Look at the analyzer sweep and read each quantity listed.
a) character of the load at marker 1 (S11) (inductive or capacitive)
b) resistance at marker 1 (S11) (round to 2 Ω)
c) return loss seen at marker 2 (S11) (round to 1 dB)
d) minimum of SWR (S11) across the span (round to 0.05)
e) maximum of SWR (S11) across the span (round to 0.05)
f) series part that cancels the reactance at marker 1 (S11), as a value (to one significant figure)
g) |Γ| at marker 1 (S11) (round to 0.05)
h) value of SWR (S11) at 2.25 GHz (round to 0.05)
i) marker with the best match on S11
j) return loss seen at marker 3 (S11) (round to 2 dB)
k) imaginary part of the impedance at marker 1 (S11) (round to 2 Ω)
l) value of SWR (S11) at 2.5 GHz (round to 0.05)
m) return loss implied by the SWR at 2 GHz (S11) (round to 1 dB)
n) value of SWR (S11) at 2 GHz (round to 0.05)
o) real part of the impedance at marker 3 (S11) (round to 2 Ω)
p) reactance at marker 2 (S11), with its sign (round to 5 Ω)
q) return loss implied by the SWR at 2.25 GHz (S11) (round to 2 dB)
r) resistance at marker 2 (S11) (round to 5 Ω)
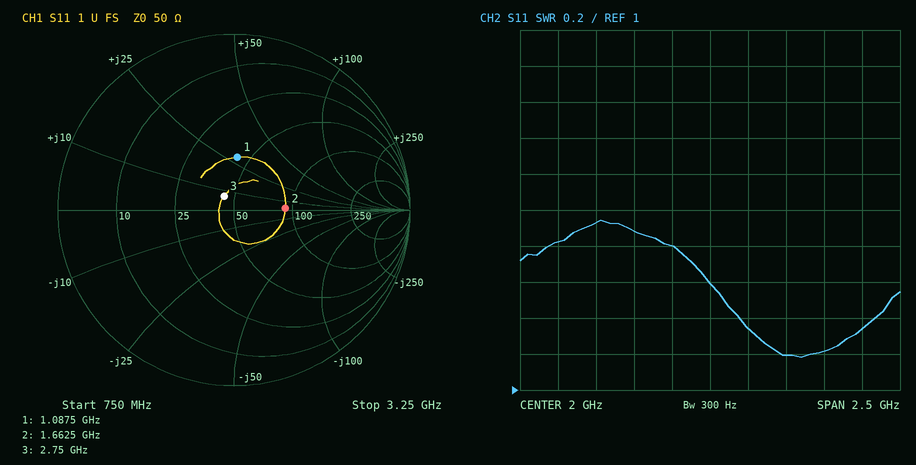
inductive
44 Ω
11 dB
1.20
1.95
5 pF
0.30
1.35
marker 3
20 dB
+28 Ω
1.20
13 dB
1.60
44 Ω
0 Ω
16 dB
90 Ω
